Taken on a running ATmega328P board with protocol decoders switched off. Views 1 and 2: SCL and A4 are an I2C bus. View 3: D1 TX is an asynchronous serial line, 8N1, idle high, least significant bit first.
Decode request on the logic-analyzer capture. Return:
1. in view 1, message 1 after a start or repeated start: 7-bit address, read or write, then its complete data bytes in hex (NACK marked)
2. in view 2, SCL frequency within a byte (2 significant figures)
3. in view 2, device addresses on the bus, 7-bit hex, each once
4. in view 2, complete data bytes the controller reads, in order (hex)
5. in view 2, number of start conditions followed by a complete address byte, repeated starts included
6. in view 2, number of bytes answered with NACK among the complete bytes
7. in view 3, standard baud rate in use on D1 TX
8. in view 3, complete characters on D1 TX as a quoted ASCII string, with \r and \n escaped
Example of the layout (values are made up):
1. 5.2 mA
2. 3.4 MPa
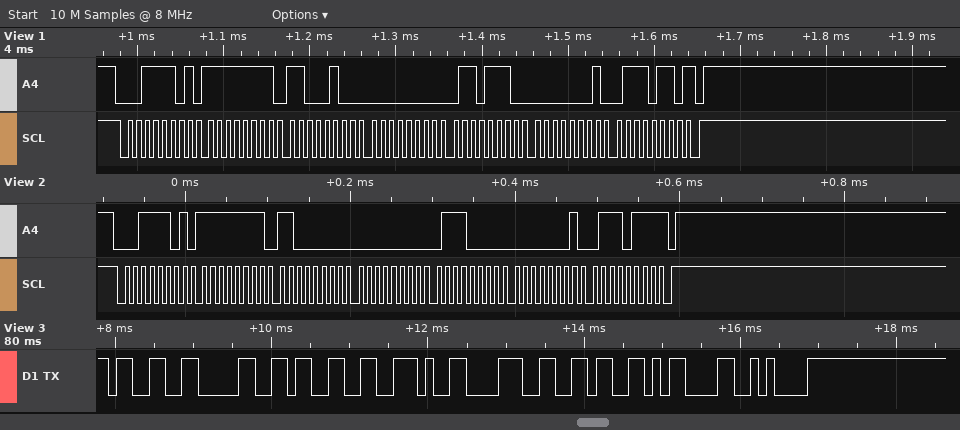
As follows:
1. 0x1E read: FF C4 00 6E 01 76 NACK
2. 100 kHz
3. 0x1E
4. FF C0 00 70 01 77
5. 1
6. 1
7. 9600 baud
8. "303.86\r\n"
